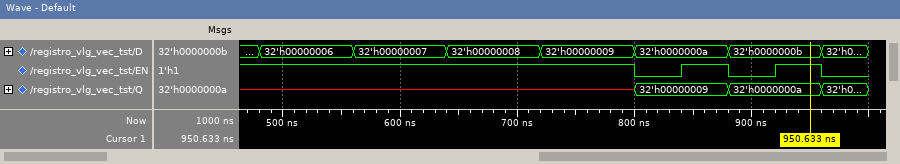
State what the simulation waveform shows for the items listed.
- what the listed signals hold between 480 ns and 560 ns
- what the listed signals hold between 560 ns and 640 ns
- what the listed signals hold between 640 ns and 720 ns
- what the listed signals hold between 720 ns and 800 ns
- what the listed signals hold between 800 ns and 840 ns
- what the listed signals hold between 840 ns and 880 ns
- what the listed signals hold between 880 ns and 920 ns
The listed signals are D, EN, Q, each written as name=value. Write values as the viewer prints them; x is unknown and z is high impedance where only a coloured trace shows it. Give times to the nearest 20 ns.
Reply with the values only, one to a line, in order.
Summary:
D=32'h00000006, EN=1, Q=x
D=32'h00000007, EN=1, Q=x
D=32'h00000008, EN=1, Q=x
D=32'h00000009, EN=1, Q=x
D=32'h0000000a, EN=0, Q=32'h00000009
D=32'h0000000a, EN=1, Q=32'h00000009
D=32'h0000000b, EN=0, Q=32'h0000000a
